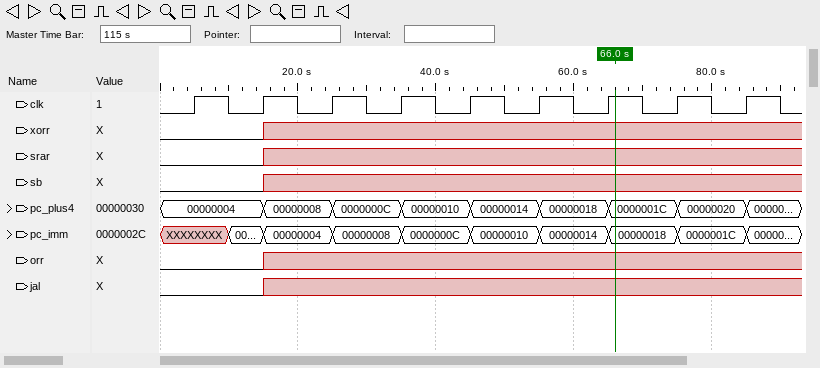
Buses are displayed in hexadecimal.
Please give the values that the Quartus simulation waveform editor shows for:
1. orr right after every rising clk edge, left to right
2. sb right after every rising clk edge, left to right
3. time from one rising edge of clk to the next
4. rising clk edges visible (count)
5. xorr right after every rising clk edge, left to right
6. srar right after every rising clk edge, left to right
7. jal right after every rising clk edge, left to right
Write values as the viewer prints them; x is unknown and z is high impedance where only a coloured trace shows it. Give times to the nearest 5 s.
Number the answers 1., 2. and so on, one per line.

1. 0 x x x x x x x x
2. 0 x x x x x x x x
3. 10 s
4. 9
5. 0 x x x x x x x x
6. 0 x x x x x x x x
7. 0 x x x x x x x x
